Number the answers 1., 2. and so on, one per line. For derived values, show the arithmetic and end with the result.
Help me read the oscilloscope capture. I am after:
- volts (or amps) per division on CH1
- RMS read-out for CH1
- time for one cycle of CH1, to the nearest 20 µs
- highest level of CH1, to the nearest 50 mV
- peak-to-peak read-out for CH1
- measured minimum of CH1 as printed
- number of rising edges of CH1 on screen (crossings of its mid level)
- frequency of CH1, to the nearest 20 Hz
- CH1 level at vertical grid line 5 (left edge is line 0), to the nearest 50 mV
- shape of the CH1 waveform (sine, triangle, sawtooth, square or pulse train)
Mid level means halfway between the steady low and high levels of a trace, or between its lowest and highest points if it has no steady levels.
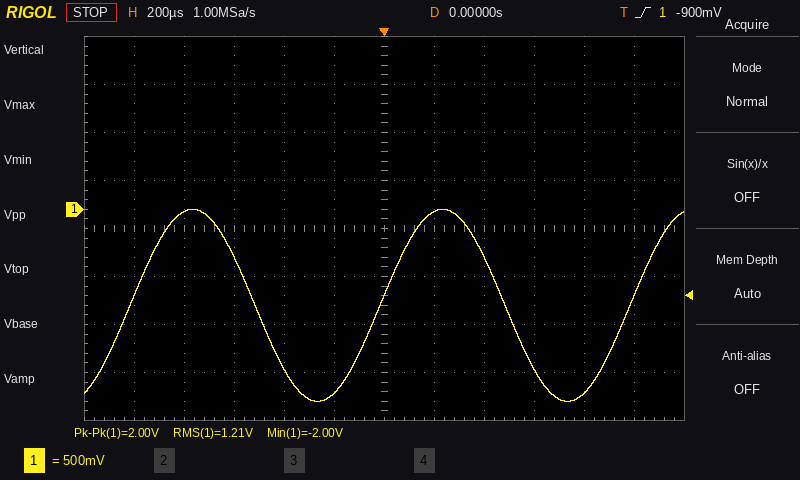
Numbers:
1. 500 mV
2. 1.21 V
3. 1.00 ms
4. 0 mV
5. 2.00 V
6. -2.00 V
7. 3
8. 1 / 1.00 ms ≈ 1.00 kHz
9. -1.90 V
10. sine
